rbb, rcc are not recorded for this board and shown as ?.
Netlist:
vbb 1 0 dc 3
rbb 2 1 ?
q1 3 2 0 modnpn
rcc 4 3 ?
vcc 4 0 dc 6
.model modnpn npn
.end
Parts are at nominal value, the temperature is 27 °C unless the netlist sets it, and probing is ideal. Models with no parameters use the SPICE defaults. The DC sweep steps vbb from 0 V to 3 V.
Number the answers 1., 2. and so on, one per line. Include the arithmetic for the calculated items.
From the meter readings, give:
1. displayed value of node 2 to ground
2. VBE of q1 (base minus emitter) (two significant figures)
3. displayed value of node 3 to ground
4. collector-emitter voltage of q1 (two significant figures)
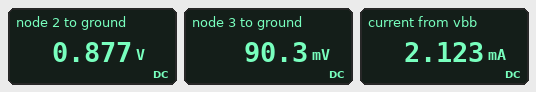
1. 0.877 V
2. 877 mV = 880 mV
3. 90.3 mV
4. 90.3 mV = 90 mV
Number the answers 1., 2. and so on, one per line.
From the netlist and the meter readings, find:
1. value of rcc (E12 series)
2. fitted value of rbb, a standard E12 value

1. 120 Ω
2. 1 kΩ
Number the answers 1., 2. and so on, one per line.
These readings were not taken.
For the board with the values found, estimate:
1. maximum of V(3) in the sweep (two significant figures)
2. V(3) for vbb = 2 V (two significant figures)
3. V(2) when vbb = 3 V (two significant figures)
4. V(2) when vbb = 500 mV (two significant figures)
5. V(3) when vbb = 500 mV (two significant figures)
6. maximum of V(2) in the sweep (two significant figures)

1. 6.0 V
2. 110 mV
3. 880 mV
4. 500 mV
5. 6.0 V
6. 880 mV
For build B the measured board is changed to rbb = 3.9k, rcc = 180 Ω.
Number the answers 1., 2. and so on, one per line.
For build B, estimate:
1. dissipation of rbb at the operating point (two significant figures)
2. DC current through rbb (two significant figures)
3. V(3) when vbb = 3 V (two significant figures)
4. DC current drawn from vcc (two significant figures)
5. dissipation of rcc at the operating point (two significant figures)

1. 1.2 mW
2. 550 µA
3. 130 mV
4. 33 mA
5. 190 mW
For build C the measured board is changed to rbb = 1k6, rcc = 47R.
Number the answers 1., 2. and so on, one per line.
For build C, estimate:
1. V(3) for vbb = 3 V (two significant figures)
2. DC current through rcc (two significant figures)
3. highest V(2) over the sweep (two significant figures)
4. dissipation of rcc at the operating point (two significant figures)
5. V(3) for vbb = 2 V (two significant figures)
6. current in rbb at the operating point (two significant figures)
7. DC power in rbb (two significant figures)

1. 190 mV
2. 120 mA
3. 900 mV
4. 720 mW
5. 2.7 V
6. 1.3 mA
7. 2.8 mW
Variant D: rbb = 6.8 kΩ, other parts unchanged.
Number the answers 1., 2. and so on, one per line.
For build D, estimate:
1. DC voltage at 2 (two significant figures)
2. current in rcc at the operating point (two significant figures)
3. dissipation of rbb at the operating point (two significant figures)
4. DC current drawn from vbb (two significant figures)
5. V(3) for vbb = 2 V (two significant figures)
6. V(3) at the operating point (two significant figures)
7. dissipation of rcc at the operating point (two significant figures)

1. 860 mV
2. 31 mA
3. 670 µW
4. 310 µA
5. 4.0 V
6. 2.2 V
7. 120 mW
